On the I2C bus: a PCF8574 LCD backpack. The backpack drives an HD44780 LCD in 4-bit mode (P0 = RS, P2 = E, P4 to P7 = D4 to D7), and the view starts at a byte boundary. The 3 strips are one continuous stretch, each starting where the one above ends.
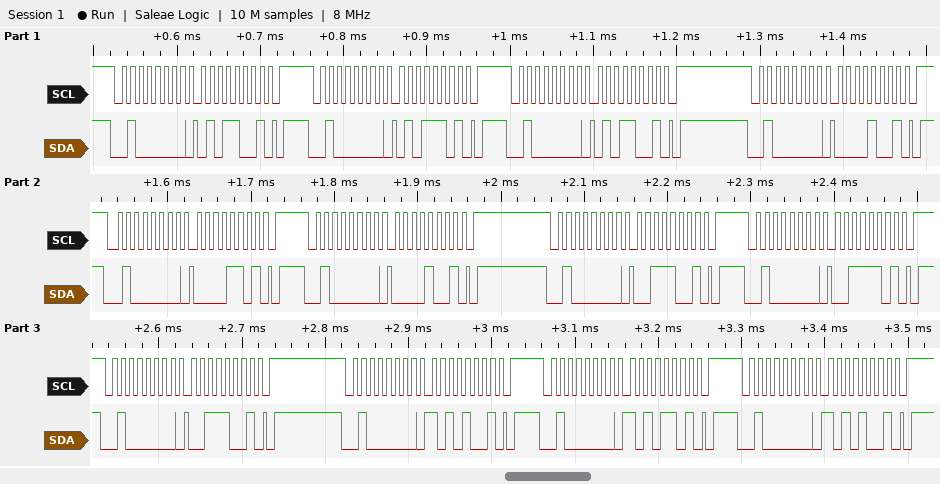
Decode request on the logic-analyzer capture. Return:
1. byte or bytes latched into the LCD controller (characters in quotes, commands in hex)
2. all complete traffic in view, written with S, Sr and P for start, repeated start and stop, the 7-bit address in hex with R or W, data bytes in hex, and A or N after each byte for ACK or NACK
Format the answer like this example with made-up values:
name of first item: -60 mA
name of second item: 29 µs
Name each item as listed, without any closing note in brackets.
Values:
byte or bytes latched into the LCD controller: 'P' ':'
all complete traffic in view, written with S, Sr and P for start, repeated start and stop, the 7-bit address in hex with R or W, data bytes in hex, and A or N after each byte for ACK or NACK: S 20W A 59 A P S 20W A 5D A P S 20W A 59 A P S 20W A 09 A P S 20W A 0D A P S 20W A 09 A P S 20W A 39 A P S 20W A 3D A P S 20W A 39 A P S 20W A A9 A P S 20W A AD A P S 20W A A9 A P
